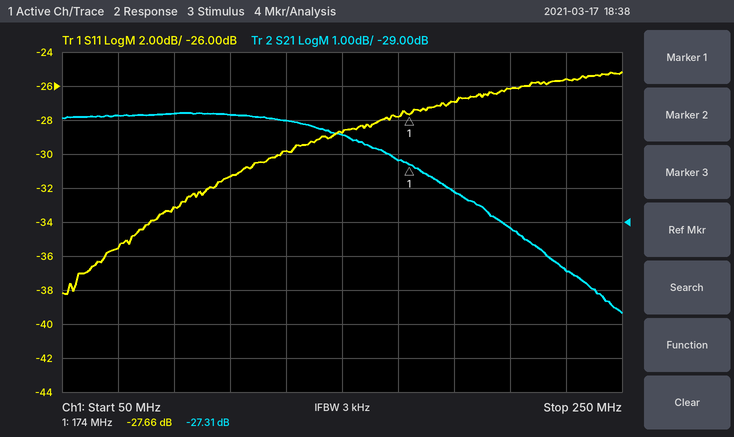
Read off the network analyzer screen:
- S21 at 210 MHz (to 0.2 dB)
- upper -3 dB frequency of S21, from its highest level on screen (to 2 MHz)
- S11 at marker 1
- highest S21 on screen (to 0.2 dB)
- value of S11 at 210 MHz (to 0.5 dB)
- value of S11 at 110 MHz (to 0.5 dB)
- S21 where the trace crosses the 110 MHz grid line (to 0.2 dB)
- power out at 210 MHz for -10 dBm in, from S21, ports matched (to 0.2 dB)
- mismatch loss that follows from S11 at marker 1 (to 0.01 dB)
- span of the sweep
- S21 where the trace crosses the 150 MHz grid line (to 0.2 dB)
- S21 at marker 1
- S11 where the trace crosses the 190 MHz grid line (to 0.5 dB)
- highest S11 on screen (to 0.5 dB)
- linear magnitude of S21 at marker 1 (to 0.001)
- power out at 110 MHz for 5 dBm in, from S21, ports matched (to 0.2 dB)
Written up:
-29.2 dB
202 MHz
-27.66 dB
-25.8 dB
-26.0 dB
-31.5 dB
-25.8 dB
-39.2 dBm
0.01 dB
200 MHz
-26.4 dB
-27.31 dB
-27.0 dB
-25.0 dB
0.043
-20.8 dBm
